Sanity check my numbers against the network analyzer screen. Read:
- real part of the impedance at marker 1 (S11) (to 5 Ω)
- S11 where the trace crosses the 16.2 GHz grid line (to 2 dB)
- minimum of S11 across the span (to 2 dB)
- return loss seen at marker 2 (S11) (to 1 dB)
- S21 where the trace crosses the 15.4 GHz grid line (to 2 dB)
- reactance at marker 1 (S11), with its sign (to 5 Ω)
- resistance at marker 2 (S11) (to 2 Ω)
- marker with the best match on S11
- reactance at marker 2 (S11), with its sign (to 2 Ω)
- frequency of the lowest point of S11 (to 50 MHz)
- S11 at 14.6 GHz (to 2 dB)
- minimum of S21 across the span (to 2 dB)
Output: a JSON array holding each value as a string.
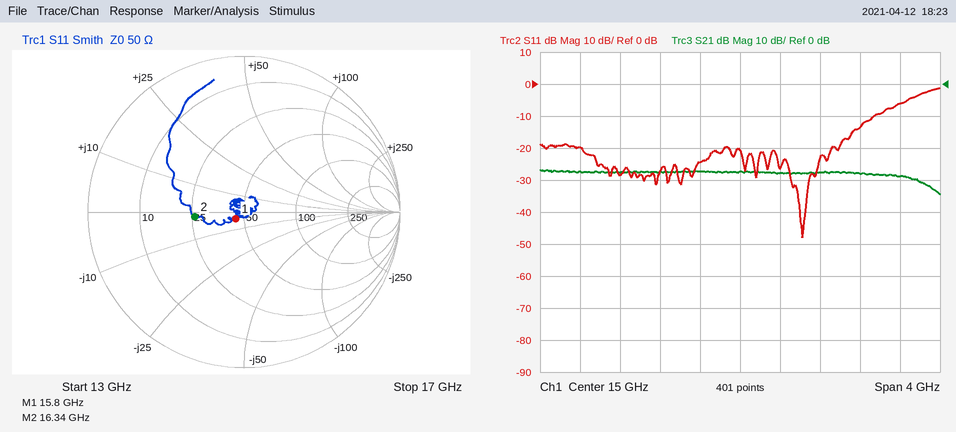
["45 Ω", "-14 dB", "-48 dB", "10 dB", "-28 dB", "-5 Ω", "26 Ω", "marker 1", "-2 Ω", "15.60 GHz", "-24 dB", "-34 dB"]
